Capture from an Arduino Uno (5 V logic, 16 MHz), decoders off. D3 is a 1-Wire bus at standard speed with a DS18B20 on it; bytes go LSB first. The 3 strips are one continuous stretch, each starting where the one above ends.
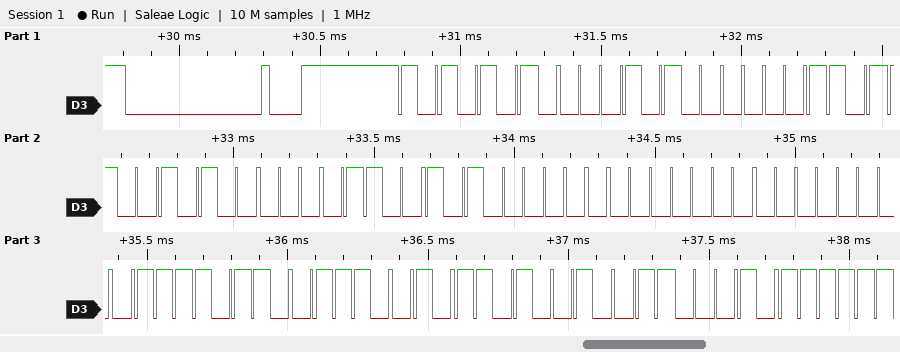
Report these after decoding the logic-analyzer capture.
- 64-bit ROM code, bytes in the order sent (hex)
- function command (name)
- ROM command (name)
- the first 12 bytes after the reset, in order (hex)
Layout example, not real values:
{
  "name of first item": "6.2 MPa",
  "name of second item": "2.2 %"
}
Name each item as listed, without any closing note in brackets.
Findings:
{
  "64-bit ROM code, bytes in the order sent": "28 B0 29 30 05 00 00 6F",
  "function command": "Write Scratchpad",
  "ROM command": "Match ROM",
  "the first 12 bytes after the reset, in order": "55 28 B0 29 30 05 00 00 6F 4E 4B 46"
}
